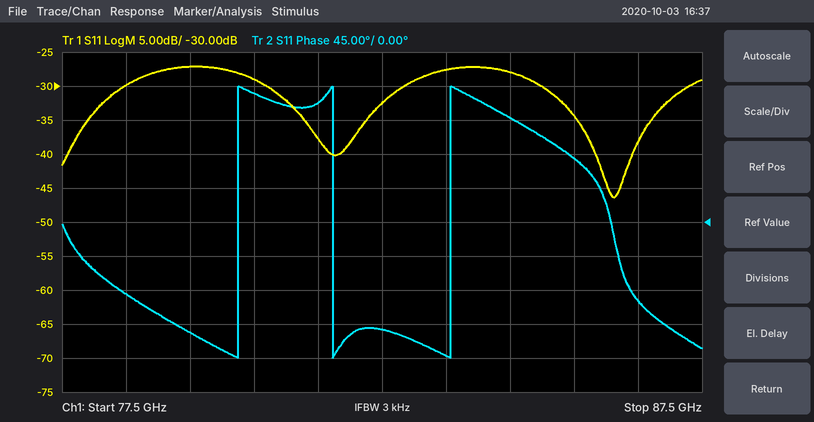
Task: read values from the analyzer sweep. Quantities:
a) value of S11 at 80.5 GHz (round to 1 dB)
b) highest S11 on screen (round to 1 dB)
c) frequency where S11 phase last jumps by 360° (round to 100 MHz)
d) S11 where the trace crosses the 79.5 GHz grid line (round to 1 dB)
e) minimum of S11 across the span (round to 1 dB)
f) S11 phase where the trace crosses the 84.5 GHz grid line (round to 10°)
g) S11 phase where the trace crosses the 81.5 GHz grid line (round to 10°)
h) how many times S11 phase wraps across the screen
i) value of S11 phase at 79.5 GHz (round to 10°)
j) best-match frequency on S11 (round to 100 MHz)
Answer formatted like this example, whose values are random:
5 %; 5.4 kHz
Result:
-29 dB; -27 dB; 83.6 GHz; -27 dB; -46 dB; 140°; 160°; 3; -150°; 86.1 GHz
